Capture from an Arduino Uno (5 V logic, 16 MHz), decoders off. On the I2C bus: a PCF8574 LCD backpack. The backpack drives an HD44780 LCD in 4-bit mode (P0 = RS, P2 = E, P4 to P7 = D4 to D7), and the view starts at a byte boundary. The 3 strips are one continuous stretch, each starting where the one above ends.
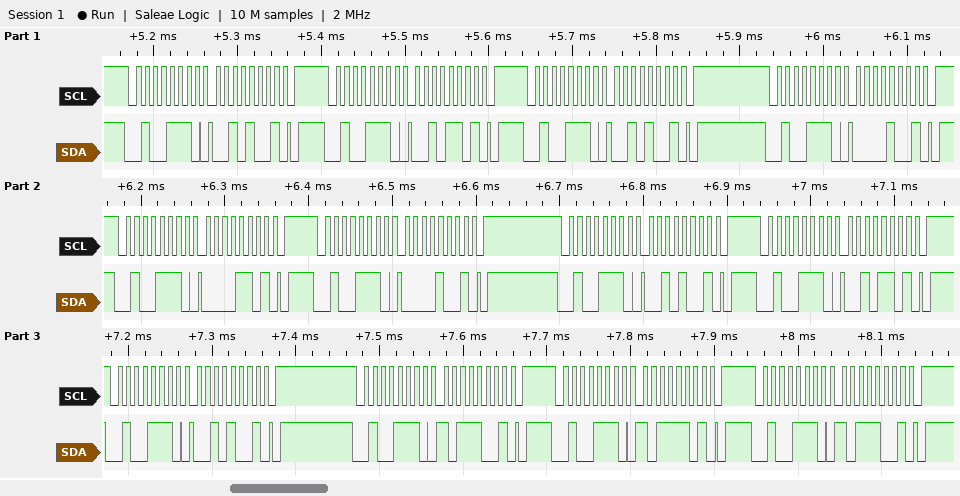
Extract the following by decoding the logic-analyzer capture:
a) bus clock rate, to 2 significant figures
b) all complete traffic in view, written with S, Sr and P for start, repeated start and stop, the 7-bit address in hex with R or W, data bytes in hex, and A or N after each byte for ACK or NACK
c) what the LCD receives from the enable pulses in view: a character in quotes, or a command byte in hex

100 kHz
S 27W A 29 A P S 27W A 2D A P S 27W A 29 A P S 27W A 09 A P S 27W A 0D A P S 27W A 09 A P S 27W A 29 A P S 27W A 2D A P S 27W A 29 A P S 27W A B9 A P S 27W A BD A P S 27W A B9 A P
' ' '+'
